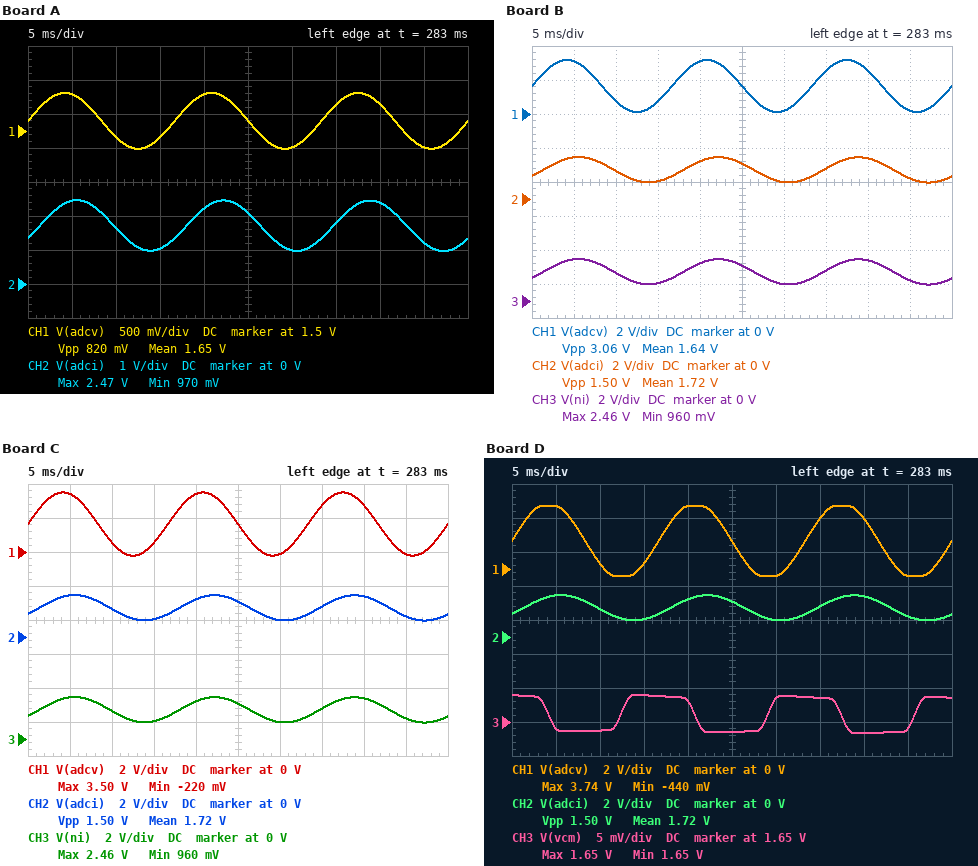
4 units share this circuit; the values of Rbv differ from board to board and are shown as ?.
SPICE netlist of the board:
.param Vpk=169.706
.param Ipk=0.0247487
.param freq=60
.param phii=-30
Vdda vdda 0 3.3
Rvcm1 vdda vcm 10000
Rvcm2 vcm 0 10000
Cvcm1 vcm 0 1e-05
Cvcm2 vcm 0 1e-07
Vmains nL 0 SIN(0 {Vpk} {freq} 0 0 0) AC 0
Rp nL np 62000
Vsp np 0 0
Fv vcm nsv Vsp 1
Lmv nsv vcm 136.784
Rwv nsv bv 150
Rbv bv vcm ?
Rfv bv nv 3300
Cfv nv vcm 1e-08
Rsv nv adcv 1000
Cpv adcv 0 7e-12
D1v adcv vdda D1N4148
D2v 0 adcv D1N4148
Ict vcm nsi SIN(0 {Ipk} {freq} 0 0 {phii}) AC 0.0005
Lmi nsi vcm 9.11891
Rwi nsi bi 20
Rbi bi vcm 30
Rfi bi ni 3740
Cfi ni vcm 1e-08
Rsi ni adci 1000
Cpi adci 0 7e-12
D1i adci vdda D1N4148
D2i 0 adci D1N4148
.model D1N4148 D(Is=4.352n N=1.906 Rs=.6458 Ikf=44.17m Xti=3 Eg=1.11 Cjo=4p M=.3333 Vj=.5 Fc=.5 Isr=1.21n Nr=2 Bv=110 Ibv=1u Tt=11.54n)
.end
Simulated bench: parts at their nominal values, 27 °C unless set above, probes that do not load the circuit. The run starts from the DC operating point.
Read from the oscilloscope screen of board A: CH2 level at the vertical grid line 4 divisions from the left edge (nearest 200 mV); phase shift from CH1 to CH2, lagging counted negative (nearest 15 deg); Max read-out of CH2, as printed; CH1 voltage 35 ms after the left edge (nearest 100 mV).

2.2 V
-30 deg
2.47 V
1.9 V
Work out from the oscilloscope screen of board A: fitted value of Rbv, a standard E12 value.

150 Ω
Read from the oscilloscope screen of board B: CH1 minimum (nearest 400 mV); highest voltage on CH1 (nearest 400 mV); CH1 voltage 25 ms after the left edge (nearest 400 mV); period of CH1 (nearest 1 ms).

0 V
3.2 V
1.6 V
17 ms
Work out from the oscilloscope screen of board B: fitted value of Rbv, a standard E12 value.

560 Ω
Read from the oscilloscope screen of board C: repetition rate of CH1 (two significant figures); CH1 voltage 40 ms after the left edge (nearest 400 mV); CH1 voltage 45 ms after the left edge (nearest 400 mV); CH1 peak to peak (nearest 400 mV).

60 Hz
2.8 V
0 V
3.6 V
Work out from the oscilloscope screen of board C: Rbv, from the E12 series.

680 Ω
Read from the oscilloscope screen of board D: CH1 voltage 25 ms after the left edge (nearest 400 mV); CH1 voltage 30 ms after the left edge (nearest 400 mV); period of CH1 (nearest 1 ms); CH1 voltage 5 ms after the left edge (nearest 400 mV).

1.6 V
-400 mV
17 ms
3.6 V
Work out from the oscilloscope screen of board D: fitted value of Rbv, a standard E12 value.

820 Ω
